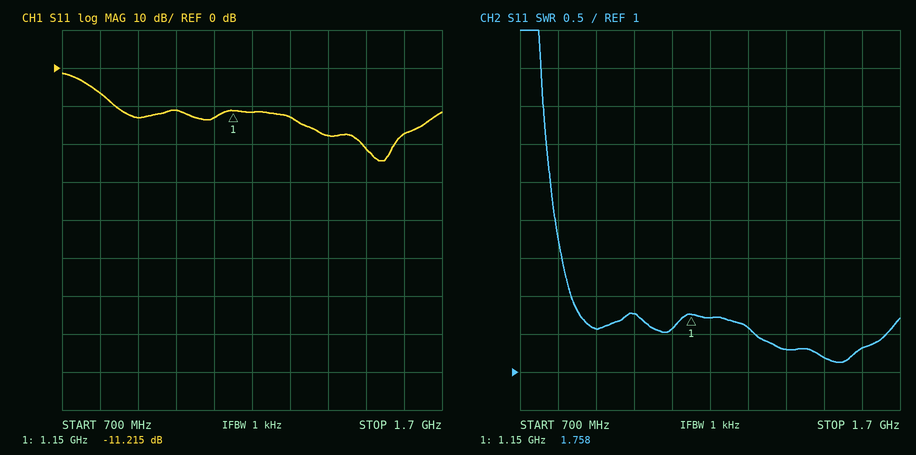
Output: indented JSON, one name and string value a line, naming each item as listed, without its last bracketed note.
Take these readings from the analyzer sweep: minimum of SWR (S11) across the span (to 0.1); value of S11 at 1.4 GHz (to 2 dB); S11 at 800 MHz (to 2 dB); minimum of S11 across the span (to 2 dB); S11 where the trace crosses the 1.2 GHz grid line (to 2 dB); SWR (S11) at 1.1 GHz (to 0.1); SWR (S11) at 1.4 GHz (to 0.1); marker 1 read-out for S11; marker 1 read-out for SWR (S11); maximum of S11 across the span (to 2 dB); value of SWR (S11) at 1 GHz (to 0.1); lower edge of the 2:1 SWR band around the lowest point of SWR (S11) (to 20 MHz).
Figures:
{
  "minimum of SWR (S11) across the span": "1.1",
  "value of S11 at 1.4 GHz": "-18 dB",
  "S11 at 800 MHz": "-6 dB",
  "minimum of S11 across the span": "-24 dB",
  "S11 where the trace crosses the 1.2 GHz grid line": "-12 dB",
  "SWR (S11) at 1.1 GHz": "1.6",
  "SWR (S11) at 1.4 GHz": "1.3",
  "marker 1 read-out for S11": "-11.215 dB",
  "marker 1 read-out for SWR": "1.758",
  "maximum of S11 across the span": "-2 dB",
  "value of SWR (S11) at 1 GHz": "1.8",
  "lower edge of the 2:1 SWR band around the lowest point of SWR (S11)": "840 MHz"
}
